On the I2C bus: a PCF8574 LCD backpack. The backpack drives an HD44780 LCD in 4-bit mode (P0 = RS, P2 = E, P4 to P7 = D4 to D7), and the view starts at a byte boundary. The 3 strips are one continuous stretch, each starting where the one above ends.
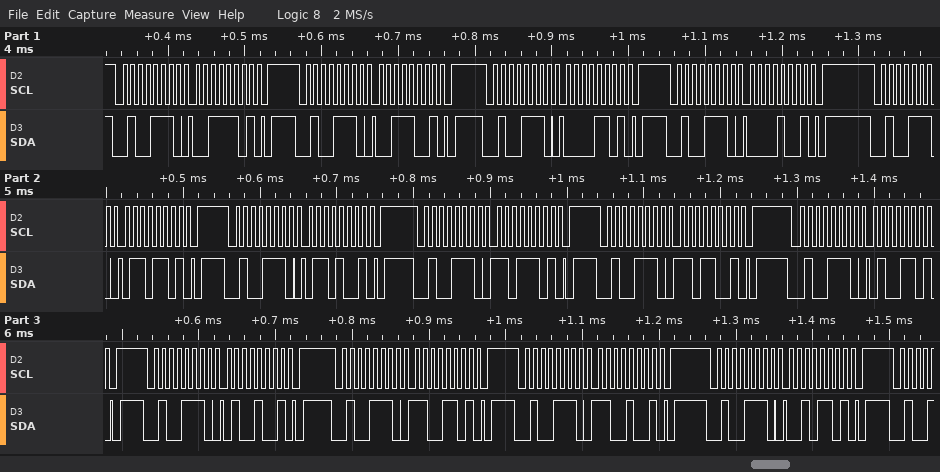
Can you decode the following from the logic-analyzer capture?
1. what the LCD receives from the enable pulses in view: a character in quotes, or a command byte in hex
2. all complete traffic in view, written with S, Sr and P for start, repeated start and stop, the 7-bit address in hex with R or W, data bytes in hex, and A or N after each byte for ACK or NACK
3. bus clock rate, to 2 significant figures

'0' 'm' 'L'
S 27W A 3D A P S 27W A 39 A P S 27W A 0D A P S 27W A 09 A P S 27W A 6D A P S 27W A 69 A P S 27W A DD A P S 27W A D9 A P S 27W A 4D A P S 27W A 49 A P S 27W A CD A P S 27W A C9 A P S 27W A 2D A P
100 kHz
